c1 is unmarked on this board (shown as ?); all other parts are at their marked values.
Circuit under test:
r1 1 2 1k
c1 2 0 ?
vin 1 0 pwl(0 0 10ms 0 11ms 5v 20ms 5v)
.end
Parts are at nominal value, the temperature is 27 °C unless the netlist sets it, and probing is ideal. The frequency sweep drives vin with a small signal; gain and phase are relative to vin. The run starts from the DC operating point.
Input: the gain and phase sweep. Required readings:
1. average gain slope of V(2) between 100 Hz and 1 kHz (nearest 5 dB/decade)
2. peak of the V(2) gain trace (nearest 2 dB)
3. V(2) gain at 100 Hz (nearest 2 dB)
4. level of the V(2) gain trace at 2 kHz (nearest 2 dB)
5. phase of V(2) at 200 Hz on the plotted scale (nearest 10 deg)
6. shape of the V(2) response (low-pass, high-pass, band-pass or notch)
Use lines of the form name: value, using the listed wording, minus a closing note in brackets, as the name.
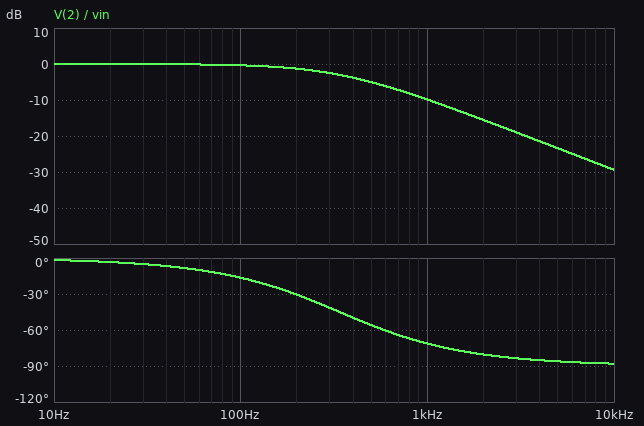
average gain slope of V(2) between 100 Hz and 1 kHz: -10 dB/decade
peak of the V(2) gain trace: 0 dB
V(2) gain at 100 Hz: 0 dB
level of the V(2) gain trace at 2 kHz: -16 dB
phase of V(2) at 200 Hz on the plotted scale: -30 deg
shape of the V(2) response: low-pass
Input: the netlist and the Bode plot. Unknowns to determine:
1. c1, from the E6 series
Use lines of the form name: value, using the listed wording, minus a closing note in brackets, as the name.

c1, from the E6 series: 470 nF
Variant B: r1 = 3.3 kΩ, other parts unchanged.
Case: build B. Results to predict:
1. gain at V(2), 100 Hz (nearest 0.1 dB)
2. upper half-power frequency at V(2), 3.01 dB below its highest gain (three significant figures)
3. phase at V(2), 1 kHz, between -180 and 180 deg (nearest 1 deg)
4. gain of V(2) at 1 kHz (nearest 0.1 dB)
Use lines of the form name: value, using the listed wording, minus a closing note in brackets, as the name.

gain at V(2), 100 Hz: -2.9 dB
upper half-power frequency at V(2), 3.01 dB below its highest gain: 103 Hz
phase at V(2), 1 kHz, between -180 and 180 deg: -84 deg
gain of V(2) at 1 kHz: -19.8 dB
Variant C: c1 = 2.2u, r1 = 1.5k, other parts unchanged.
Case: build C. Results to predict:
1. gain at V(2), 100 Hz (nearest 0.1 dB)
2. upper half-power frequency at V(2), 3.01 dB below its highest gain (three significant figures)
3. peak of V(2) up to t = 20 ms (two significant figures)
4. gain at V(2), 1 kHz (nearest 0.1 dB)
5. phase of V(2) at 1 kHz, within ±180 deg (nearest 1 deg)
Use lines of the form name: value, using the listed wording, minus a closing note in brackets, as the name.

gain at V(2), 100 Hz: -7.2 dB
upper half-power frequency at V(2), 3.01 dB below its highest gain: 48.2 Hz
peak of V(2) up to t = 20 ms: 4.7 V
gain at V(2), 1 kHz: -26.3 dB
phase of V(2) at 1 kHz, within ±180 deg: -87 deg
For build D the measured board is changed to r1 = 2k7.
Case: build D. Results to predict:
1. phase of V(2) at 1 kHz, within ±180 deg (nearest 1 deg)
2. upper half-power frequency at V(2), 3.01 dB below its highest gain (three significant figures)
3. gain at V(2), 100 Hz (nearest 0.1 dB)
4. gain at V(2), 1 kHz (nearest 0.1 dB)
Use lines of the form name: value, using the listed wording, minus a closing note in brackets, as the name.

phase of V(2) at 1 kHz, within ±180 deg: -83 deg
upper half-power frequency at V(2), 3.01 dB below its highest gain: 125 Hz
gain at V(2), 100 Hz: -2.1 dB
gain at V(2), 1 kHz: -18.1 dB
